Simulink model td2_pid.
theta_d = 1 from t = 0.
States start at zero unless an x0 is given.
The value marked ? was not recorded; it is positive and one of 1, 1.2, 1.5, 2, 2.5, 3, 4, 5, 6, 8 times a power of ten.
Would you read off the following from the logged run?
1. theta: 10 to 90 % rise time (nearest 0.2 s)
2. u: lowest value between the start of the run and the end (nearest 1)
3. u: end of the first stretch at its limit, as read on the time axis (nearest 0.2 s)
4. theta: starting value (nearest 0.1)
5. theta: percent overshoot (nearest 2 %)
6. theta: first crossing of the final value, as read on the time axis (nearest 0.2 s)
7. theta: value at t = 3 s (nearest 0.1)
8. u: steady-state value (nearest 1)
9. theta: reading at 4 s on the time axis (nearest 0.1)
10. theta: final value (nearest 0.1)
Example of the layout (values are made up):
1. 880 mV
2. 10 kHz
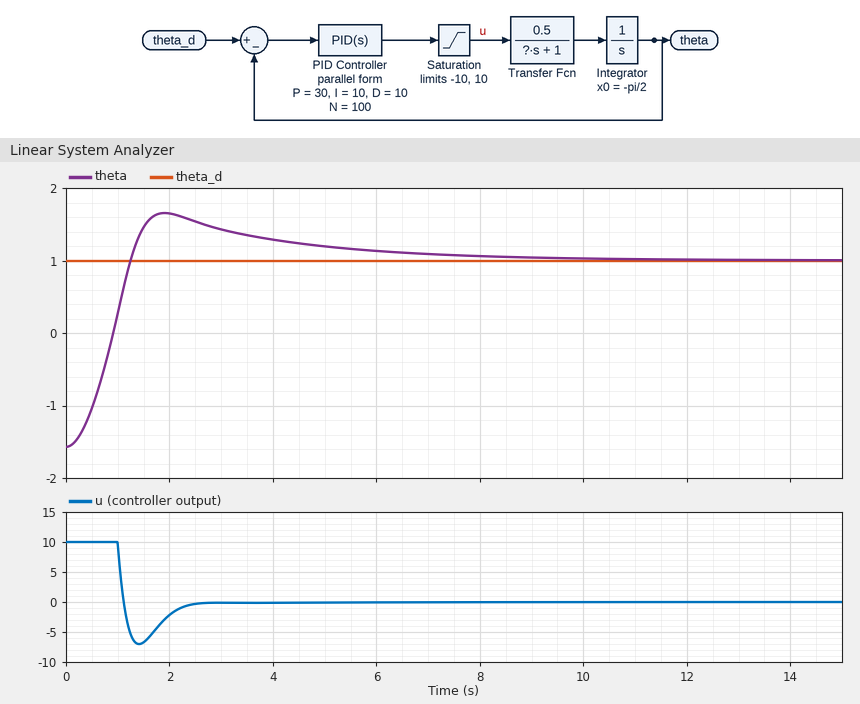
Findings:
1. 0.8 s
2. -7
3. 1.0 s
4. -1.6
5. 26 %
6. 1.2 s
7. 1.4
8. 0
9. 1.3
10. 1.0
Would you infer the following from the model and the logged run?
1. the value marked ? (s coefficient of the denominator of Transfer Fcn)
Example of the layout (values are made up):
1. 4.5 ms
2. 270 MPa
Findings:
1. 1
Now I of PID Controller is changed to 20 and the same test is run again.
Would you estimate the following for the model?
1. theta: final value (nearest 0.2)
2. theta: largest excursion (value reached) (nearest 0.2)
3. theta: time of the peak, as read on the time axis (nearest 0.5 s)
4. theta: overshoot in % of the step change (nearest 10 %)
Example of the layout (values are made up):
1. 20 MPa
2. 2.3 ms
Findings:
1. 1.0
2. 2.2
3. 2.0 s
4. 50 %
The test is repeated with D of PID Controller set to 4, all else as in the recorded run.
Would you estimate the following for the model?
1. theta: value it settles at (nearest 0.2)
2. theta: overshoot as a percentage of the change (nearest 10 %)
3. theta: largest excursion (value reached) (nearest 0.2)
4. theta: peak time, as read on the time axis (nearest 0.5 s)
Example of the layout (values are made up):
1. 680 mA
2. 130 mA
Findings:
1. 1.0
2. 40 %
3. 2.2
4. 2.0 s
